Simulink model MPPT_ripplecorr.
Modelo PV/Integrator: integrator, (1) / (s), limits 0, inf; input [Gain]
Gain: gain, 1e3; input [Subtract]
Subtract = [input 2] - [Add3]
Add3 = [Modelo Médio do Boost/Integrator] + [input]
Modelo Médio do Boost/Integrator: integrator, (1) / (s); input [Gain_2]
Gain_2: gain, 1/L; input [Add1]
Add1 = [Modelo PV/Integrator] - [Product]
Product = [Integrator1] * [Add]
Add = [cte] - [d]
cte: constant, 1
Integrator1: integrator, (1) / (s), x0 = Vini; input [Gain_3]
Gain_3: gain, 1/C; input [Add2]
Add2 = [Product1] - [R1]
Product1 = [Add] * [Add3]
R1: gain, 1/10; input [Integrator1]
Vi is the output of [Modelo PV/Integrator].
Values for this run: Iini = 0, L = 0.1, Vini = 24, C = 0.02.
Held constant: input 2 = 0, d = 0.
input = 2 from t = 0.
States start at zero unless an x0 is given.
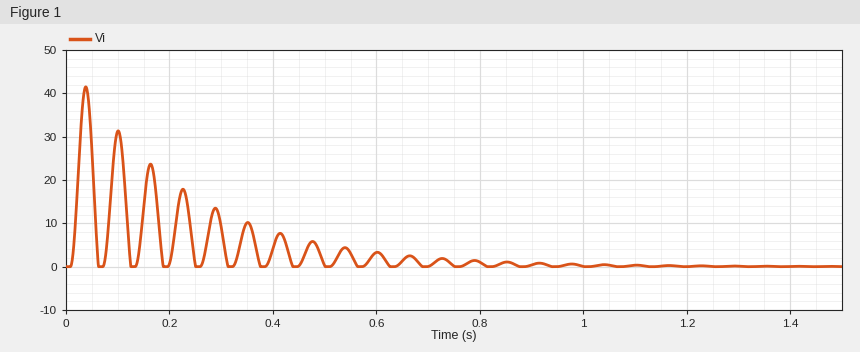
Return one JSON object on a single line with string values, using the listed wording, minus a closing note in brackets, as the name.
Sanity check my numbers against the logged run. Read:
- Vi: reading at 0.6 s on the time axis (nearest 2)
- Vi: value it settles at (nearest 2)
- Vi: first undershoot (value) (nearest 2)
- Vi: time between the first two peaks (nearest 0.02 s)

{"Vi: reading at 0.6 s on the time axis": "4", "Vi: value it settles at": "0", "Vi: first undershoot (value)": "0", "Vi: time between the first two peaks": "0.06 s"}
